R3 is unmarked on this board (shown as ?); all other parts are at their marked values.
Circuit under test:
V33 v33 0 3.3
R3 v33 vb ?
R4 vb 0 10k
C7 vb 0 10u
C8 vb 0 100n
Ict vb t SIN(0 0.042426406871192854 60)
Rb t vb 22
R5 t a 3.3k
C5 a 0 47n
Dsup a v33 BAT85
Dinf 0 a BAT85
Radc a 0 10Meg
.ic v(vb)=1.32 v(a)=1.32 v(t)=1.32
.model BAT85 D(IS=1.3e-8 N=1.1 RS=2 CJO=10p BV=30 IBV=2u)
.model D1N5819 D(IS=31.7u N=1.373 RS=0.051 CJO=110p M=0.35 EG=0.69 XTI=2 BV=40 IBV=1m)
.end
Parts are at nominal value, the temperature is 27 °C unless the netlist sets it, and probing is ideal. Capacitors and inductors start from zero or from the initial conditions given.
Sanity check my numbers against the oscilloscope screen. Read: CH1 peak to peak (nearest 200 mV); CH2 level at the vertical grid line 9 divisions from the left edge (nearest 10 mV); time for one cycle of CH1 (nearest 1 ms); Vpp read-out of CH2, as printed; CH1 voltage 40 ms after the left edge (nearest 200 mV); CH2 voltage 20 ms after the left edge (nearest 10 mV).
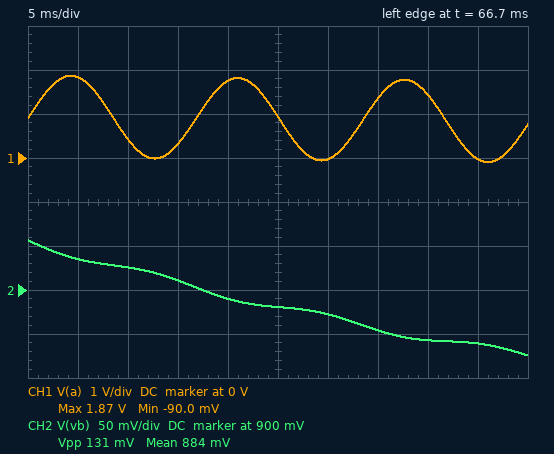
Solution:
2.0 V
840 mV
17 ms
131 mV
1.4 V
890 mV
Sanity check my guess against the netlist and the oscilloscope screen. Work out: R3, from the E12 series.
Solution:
39 kΩ
